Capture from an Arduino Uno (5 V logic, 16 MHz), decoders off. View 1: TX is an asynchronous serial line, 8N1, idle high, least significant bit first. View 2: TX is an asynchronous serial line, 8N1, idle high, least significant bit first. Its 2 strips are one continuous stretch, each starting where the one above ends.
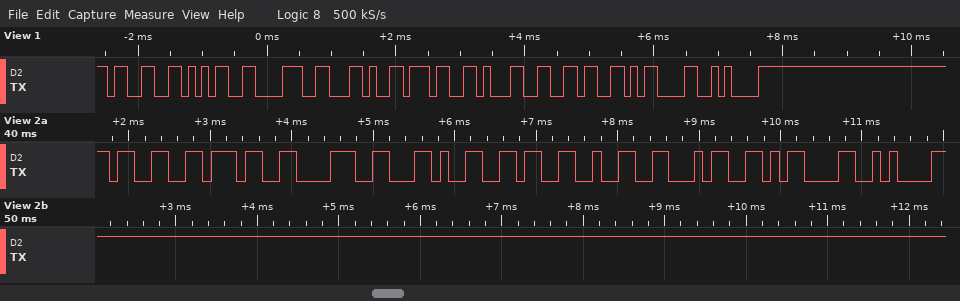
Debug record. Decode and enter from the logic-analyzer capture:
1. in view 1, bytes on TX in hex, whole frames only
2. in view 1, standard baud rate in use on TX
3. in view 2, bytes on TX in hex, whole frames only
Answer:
0x33 0x35 0x38 0x2C 0x37 0x31 0x36 0x0D 0x0A
9600 baud
0x33 0x37 0x38 0x2C 0x36 0x32 0x34 0x0D 0x0A
